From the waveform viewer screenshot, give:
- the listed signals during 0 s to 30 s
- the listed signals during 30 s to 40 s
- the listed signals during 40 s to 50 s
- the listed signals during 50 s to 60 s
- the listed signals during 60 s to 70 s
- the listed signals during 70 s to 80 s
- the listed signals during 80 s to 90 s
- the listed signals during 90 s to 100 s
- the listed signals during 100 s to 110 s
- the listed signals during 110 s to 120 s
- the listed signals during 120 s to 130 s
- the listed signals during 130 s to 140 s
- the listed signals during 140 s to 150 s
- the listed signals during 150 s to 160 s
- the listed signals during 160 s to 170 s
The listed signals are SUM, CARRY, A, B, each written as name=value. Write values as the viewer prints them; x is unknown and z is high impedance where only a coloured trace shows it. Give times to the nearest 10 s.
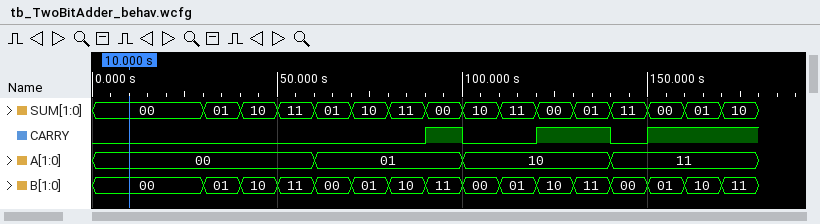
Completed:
SUM=00, CARRY=0, A=00, B=00
SUM=01, CARRY=0, A=00, B=01
SUM=10, CARRY=0, A=00, B=10
SUM=11, CARRY=0, A=00, B=11
SUM=01, CARRY=0, A=01, B=00
SUM=10, CARRY=0, A=01, B=01
SUM=11, CARRY=0, A=01, B=10
SUM=00, CARRY=1, A=01, B=11
SUM=10, CARRY=0, A=10, B=00
SUM=11, CARRY=0, A=10, B=01
SUM=00, CARRY=1, A=10, B=10
SUM=01, CARRY=1, A=10, B=11
SUM=11, CARRY=0, A=11, B=00
SUM=00, CARRY=1, A=11, B=01
SUM=01, CARRY=1, A=11, B=10
